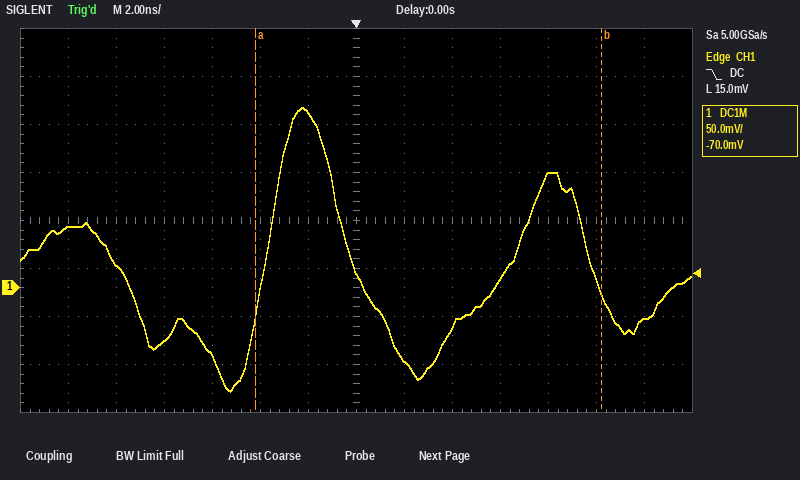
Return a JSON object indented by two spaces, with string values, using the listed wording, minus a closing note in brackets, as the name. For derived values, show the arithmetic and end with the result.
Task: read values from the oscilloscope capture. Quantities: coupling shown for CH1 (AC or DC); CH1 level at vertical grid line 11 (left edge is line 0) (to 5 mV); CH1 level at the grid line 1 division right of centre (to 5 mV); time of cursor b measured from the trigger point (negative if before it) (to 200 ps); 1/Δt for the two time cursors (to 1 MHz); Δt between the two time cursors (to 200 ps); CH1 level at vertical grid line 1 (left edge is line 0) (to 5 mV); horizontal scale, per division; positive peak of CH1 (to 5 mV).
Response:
{
  "coupling shown for CH1": "DC",
  "CH1 level at vertical grid line 11 (left edge is line 0)": "120 mV",
  "CH1 level at the grid line 1 division right of centre": "-75 mV",
  "time of cursor b measured from the trigger point (negative if before it)": "+10.2 ns",
  "1/Δt for the two time cursors": "1 / 14.4 ns ≈ 69 MHz",
  "Δt between the two time cursors": "14.4 ns",
  "CH1 level at vertical grid line 1 (left edge is line 0)": "65 mV",
  "horizontal scale, per division": "2 ns",
  "positive peak of CH1": "190 mV"
}
